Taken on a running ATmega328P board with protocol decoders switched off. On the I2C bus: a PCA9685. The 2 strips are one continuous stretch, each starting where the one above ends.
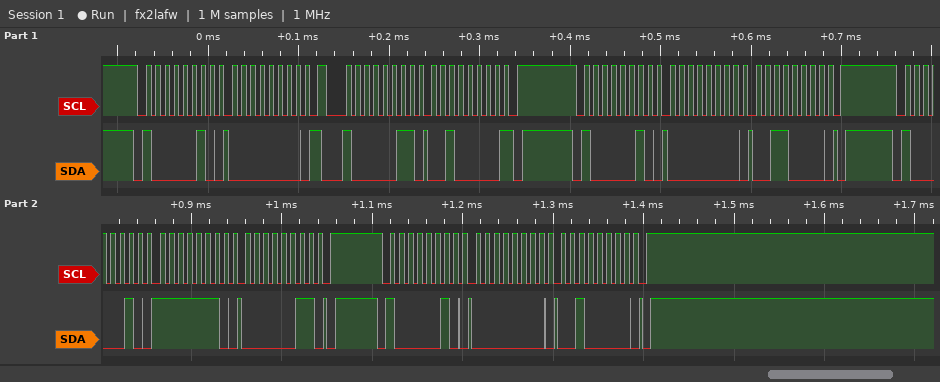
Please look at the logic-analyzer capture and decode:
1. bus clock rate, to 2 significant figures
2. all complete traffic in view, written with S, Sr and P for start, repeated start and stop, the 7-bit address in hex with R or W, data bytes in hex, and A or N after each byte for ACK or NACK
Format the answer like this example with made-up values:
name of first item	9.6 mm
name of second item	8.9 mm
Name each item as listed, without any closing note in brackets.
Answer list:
bus clock rate, to 2 significant figures	100 kHz
all complete traffic in view, written with S, Sr and P for start, repeated start and stop, the 7-bit address in hex with R or W, data bytes in hex, and A or N after each byte for ACK or NACK	S 41W A 00 A Sr 41R A 20 N P S 41W A 00 A 30 A P S 41W A FE A 03 A P S 41W A 00 A 20 A P
